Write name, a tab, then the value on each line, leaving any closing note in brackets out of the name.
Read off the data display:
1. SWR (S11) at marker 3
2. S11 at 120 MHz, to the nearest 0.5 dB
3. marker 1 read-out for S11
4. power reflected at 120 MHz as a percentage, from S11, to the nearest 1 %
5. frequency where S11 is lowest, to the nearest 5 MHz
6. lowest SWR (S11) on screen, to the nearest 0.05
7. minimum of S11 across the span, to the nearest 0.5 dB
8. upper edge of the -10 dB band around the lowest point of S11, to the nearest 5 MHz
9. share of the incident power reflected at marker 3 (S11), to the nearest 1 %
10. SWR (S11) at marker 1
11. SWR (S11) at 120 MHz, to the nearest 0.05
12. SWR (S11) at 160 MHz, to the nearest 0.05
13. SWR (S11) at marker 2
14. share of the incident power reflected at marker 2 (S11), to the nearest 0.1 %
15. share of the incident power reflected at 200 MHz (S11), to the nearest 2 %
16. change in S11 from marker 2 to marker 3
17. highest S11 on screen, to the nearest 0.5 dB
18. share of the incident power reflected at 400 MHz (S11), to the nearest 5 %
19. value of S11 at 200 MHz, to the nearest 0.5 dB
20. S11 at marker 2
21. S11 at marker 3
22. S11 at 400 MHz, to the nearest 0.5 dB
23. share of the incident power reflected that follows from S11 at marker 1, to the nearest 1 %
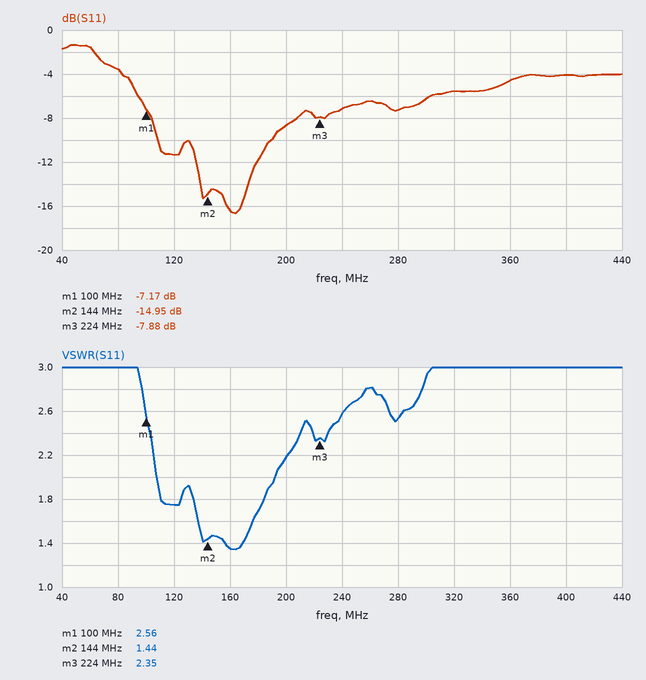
SWR (S11) at marker 3	2.35
S11 at 120 MHz, to the nearest 0.5 dB	-11.5 dB
marker 1 read-out for S11	-7.17 dB
power reflected at 120 MHz as a percentage, from S11, to the nearest 1 %	7 %
frequency where S11 is lowest, to the nearest 5 MHz	165 MHz
lowest SWR (S11) on screen, to the nearest 0.05	1.35
minimum of S11 across the span, to the nearest 0.5 dB	-16.5 dB
upper edge of the -10 dB band around the lowest point of S11, to the nearest 5 MHz	190 MHz
share of the incident power reflected at marker 3 (S11), to the nearest 1 %	16 %
SWR (S11) at marker 1	2.56
SWR (S11) at 120 MHz, to the nearest 0.05	1.75
SWR (S11) at 160 MHz, to the nearest 0.05	1.35
SWR (S11) at marker 2	1.44
share of the incident power reflected at marker 2 (S11), to the nearest 0.1 %	3.2 %
share of the incident power reflected at 200 MHz (S11), to the nearest 2 %	14 %
change in S11 from marker 2 to marker 3	7.07 dB
highest S11 on screen, to the nearest 0.5 dB	-1.5 dB
share of the incident power reflected at 400 MHz (S11), to the nearest 5 %	40 %
value of S11 at 200 MHz, to the nearest 0.5 dB	-8.5 dB
S11 at marker 2	-14.95 dB
S11 at marker 3	-7.88 dB
S11 at 400 MHz, to the nearest 0.5 dB	-4.0 dB
share of the incident power reflected that follows from S11 at marker 1, to the nearest 1 %	19 %
